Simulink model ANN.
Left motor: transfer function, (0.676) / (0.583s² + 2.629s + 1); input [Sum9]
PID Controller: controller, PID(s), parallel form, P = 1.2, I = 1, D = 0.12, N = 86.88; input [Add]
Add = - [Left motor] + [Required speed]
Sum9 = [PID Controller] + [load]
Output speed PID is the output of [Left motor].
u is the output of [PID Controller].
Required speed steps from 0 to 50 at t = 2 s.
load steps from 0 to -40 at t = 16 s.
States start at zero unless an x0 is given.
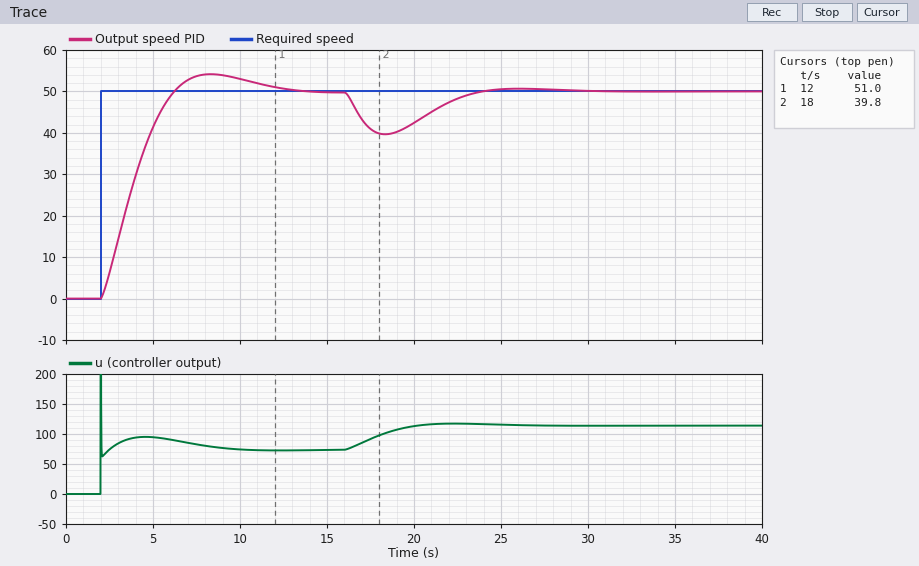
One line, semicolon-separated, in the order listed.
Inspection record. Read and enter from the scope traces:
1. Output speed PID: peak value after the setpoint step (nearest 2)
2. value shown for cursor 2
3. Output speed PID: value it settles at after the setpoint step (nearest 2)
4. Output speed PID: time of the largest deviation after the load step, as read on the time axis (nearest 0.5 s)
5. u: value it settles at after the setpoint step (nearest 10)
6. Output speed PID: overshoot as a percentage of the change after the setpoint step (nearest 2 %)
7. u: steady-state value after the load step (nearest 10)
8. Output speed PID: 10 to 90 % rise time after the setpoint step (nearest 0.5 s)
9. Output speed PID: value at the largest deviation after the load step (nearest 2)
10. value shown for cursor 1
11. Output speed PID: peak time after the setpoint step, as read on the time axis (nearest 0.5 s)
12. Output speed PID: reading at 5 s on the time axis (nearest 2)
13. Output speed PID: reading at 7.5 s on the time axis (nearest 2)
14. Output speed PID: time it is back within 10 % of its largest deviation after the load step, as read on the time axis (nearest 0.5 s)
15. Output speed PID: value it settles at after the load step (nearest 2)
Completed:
54; 39.8; 50; 18.5 s; 70; 8 %; 110; 3.0 s; 40; 51.0; 8.5 s; 42; 54; 23.0 s; 50
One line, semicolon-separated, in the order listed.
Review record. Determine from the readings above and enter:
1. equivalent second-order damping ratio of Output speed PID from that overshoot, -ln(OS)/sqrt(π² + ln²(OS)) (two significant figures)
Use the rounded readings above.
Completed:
0.63
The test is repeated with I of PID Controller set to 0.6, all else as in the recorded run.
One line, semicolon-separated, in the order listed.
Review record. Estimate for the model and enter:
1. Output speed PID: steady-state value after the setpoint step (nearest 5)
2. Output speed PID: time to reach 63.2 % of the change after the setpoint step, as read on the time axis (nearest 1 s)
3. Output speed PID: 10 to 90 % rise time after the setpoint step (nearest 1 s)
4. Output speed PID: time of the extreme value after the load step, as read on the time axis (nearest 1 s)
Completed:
50; 5 s; 5 s; 19 s
